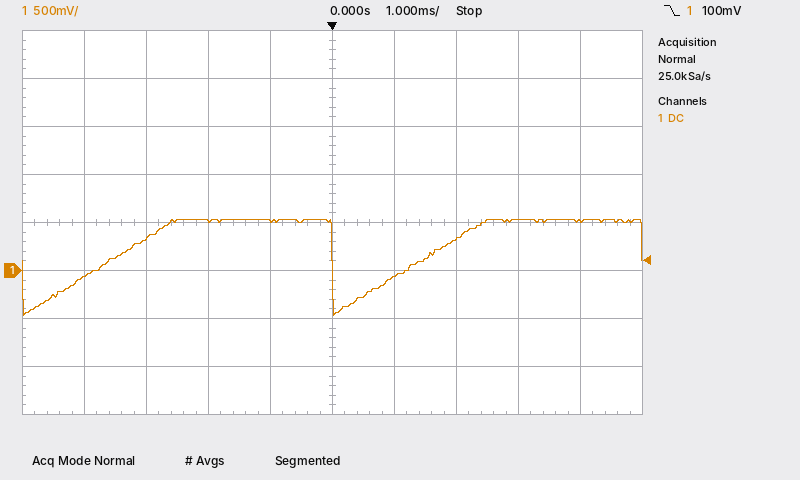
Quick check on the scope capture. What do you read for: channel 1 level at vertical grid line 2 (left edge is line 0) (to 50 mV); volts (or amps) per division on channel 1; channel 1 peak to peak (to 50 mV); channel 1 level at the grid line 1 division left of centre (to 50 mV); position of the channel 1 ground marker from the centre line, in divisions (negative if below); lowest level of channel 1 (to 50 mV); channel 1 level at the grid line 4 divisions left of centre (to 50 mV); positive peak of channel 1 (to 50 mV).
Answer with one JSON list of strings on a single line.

["350 mV", "500 mV", "1.00 V", "500 mV", "-1.0 div", "-450 mV", "-50 mV", "550 mV"]
